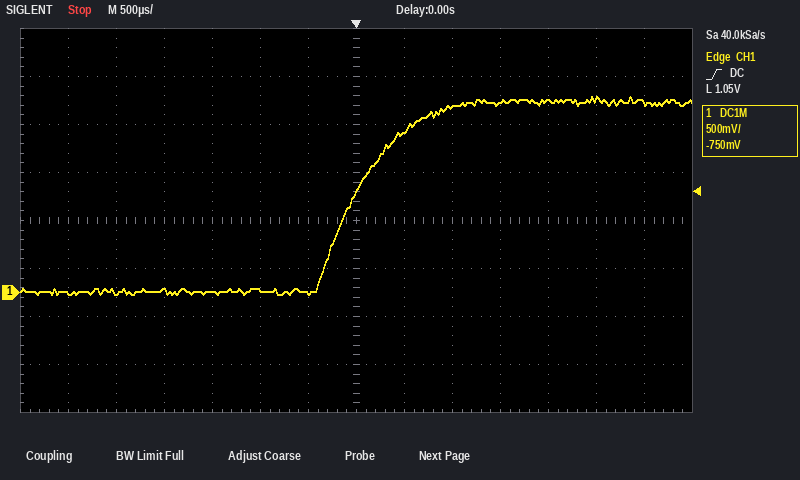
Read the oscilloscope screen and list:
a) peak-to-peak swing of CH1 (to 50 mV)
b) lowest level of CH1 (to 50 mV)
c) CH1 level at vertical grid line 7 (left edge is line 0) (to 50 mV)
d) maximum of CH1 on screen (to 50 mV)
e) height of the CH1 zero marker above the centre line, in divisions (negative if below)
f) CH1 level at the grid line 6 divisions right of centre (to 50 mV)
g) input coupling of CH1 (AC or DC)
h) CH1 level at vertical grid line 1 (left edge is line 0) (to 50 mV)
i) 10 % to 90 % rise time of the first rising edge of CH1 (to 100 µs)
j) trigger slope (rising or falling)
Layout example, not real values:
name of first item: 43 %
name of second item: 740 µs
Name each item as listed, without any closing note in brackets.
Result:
peak-to-peak swing of CH1: 2.05 V
lowest level of CH1: 0 mV
CH1 level at vertical grid line 7 (left edge is line 0): 1.05 V
maximum of CH1 on screen: 2.05 V
height of the CH1 zero marker above the centre line, in divisions: -1.5 div
CH1 level at the grid line 6 divisions right of centre: 2.00 V
input coupling of CH1: DC
CH1 level at vertical grid line 1 (left edge is line 0): 0 mV
10 % to 90 % rise time of the first rising edge of CH1: 1.0 ms
trigger slope: rising
